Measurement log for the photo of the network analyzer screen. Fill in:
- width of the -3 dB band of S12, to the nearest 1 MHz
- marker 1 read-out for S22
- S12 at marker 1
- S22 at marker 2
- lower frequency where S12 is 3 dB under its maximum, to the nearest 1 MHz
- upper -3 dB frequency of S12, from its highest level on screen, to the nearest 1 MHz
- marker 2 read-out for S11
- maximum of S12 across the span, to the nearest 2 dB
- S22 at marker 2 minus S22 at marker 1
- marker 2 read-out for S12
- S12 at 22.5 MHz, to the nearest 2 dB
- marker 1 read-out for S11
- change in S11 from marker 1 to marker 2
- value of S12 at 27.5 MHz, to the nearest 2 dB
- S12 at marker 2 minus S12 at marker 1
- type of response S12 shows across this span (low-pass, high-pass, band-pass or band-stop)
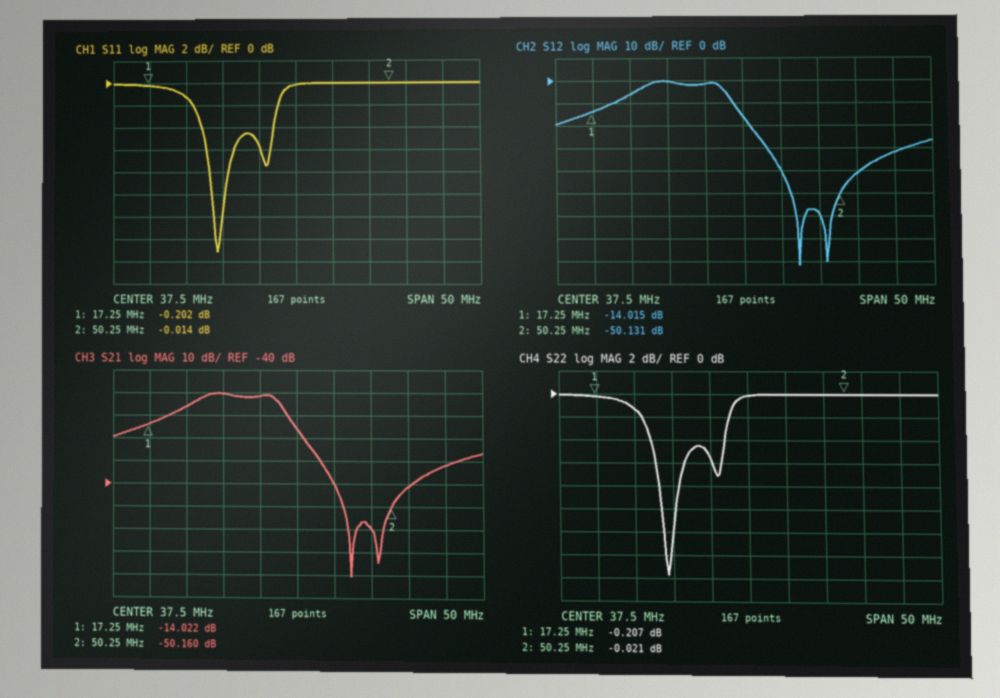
11 MHz
-0.207 dB
-14.015 dB
-0.021 dB
24 MHz
35 MHz
-0.014 dB
0 dB
0.186 dB
-50.131 dB
-6 dB
-0.202 dB
0.188 dB
0 dB
-36.116 dB
band-pass
